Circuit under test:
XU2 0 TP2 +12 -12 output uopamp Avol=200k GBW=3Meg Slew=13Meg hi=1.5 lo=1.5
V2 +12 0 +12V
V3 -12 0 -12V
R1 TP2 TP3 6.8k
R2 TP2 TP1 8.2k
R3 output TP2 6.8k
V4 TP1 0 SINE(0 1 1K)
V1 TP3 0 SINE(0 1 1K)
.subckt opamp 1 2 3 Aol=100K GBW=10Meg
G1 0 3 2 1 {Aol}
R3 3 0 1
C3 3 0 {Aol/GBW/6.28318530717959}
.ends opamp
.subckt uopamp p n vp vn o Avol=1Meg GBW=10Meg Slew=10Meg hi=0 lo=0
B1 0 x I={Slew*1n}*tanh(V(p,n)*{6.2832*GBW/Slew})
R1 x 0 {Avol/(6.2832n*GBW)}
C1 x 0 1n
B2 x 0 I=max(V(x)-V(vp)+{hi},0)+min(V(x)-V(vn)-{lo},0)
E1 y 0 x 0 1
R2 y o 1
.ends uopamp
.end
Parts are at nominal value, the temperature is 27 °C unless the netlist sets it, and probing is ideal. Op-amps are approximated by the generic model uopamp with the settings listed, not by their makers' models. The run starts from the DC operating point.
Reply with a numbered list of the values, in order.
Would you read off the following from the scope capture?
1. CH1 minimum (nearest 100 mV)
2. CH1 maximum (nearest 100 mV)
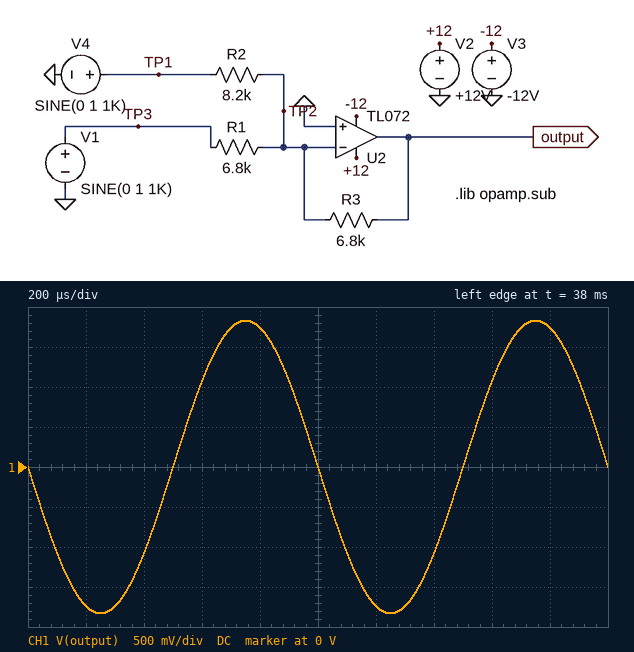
1. -1.8 V
2. 1.8 V
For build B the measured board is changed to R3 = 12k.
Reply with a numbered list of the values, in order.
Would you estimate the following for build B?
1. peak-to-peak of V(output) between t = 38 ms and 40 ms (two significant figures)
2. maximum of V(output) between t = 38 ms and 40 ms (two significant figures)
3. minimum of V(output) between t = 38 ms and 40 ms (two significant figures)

1. 6.5 V
2. 3.2 V
3. -3.2 V
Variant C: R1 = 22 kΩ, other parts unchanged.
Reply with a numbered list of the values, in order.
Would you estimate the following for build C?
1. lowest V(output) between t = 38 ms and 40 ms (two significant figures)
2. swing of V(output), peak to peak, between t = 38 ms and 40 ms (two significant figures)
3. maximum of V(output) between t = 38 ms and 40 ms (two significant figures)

1. -1.1 V
2. 2.3 V
3. 1.1 V
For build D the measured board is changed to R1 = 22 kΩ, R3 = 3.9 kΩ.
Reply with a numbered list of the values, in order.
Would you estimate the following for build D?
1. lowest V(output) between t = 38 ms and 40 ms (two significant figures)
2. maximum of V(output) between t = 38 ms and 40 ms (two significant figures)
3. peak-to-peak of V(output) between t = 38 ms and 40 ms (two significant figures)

1. -650 mV
2. 650 mV
3. 1.3 V
